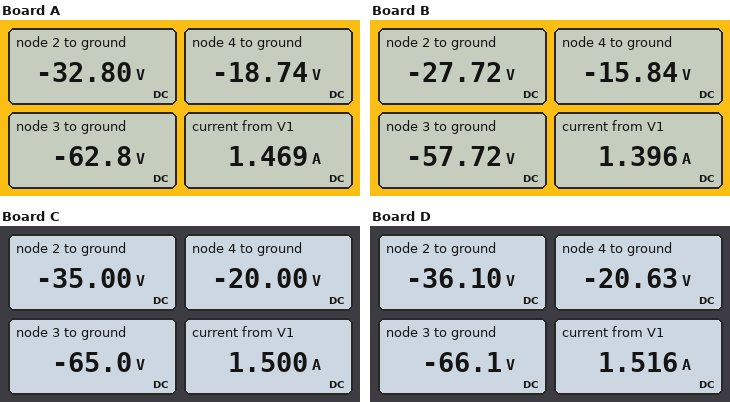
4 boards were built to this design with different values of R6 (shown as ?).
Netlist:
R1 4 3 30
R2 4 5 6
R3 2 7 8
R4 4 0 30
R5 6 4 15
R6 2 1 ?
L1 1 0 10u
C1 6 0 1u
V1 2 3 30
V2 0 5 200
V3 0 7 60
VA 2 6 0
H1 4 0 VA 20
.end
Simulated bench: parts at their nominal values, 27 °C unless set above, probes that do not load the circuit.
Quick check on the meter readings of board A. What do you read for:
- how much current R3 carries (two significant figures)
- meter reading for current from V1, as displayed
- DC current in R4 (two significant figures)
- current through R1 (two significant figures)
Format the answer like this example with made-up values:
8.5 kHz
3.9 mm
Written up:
3.4 A
1.469 A
620 mA
1.5 A
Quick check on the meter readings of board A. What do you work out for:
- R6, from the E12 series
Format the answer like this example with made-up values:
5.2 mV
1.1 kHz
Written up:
33 Ω
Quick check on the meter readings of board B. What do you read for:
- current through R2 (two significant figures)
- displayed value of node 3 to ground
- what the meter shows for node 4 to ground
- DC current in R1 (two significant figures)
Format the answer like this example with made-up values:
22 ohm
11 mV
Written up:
31 A
-57.72 V
-15.84 V
1.4 A
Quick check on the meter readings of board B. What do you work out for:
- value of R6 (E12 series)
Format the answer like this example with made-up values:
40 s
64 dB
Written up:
15 Ω
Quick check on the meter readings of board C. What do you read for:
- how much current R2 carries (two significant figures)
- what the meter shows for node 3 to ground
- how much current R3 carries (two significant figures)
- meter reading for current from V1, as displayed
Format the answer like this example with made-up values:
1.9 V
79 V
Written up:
30 A
-65.0 V
3.1 A
1.500 A
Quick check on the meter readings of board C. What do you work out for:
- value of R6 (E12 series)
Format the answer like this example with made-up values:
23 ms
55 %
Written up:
56 Ω
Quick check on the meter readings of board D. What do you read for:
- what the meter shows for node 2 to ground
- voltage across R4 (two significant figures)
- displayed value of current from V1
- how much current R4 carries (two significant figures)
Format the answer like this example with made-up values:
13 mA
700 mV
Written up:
-36.10 V
21 V
1.516 A
690 mA
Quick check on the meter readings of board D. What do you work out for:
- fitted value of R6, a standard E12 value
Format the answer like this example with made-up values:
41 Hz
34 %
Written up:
82 Ω
